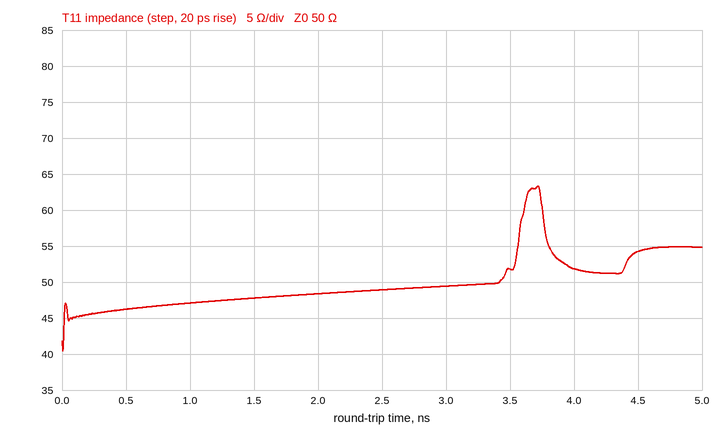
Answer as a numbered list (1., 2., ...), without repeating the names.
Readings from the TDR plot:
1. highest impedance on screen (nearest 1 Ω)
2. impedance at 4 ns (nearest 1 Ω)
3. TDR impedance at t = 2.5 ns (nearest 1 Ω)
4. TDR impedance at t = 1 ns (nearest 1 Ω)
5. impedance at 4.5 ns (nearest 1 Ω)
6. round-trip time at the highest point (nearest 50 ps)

1. 63 Ω
2. 52 Ω
3. 49 Ω
4. 47 Ω
5. 54 Ω
6. 3.70 ns
